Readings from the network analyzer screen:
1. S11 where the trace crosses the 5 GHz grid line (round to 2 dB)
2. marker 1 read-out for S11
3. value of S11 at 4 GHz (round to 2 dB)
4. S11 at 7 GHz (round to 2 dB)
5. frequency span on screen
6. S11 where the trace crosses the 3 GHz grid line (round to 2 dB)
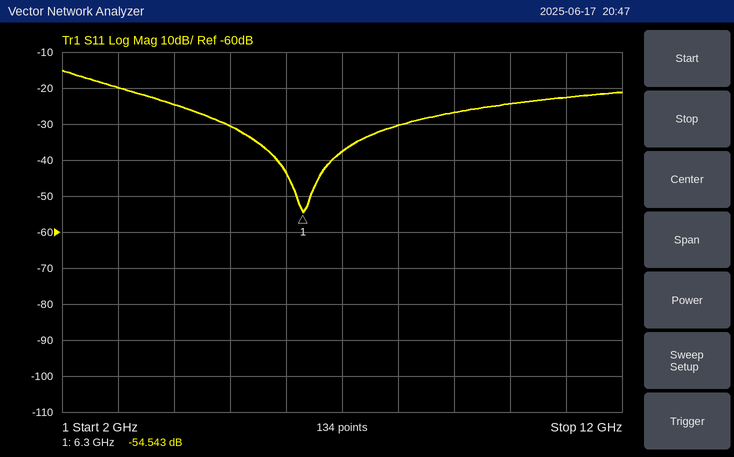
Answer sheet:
-30 dB
-54.543 dB
-24 dB
-38 dB
10 GHz
-20 dB
